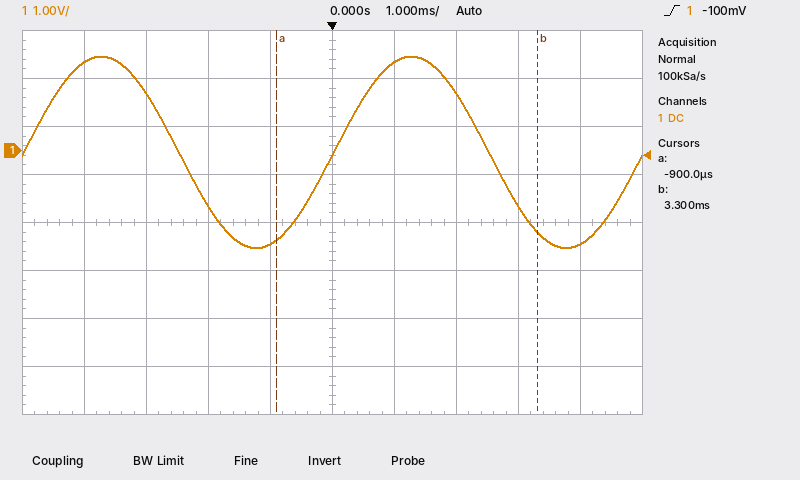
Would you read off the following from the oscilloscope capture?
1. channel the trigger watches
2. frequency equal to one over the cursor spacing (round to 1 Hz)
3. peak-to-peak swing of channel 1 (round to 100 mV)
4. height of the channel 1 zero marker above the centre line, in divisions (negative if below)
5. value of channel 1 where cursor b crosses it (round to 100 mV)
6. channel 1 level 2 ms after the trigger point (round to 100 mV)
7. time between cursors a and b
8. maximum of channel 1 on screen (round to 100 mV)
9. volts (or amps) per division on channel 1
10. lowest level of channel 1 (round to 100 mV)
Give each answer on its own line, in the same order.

channel 1
238 Hz
4.0 V
+1.5 div
-1.7 V
1.2 V
4.2 ms
2.0 V
1 V
-2.0 V
